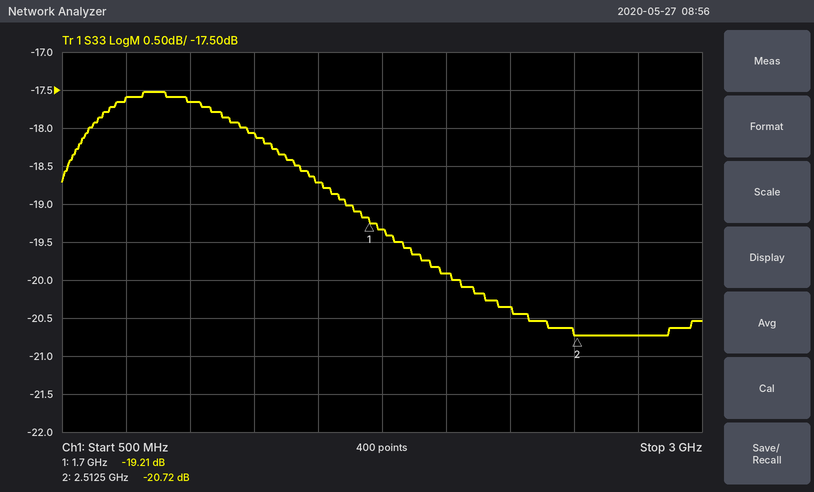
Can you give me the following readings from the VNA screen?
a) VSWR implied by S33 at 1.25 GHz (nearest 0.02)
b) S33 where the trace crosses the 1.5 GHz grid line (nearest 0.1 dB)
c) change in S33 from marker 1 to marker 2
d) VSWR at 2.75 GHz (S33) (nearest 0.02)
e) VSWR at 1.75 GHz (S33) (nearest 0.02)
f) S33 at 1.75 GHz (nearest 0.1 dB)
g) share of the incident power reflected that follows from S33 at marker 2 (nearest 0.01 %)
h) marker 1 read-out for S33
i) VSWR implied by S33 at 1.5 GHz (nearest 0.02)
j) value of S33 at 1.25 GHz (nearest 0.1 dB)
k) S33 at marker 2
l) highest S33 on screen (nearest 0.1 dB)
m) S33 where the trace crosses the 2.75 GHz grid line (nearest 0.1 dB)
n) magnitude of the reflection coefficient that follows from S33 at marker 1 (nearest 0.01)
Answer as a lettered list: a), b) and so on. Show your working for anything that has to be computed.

a) |Γ| = 10^(-18.1/20) = 0.1245; VSWR = (1 + 0.1245)/(1 − 0.1245) ≈ 1.28
b) -18.7 dB
c) -20.72 − (-19.21) = -1.51 dB
d) |Γ| = 10^(-20.7/20) = 0.0923; VSWR = (1 + 0.0923)/(1 − 0.0923) ≈ 1.20
e) |Γ| = 10^(-19.3/20) = 0.1084; VSWR = (1 + 0.1084)/(1 − 0.1084) ≈ 1.24
f) -19.3 dB
g) 10^(-20.72/10) ≈ 0.85 %
h) -19.21 dB
i) |Γ| = 10^(-18.7/20) = 0.1161; VSWR = (1 + 0.1161)/(1 − 0.1161) ≈ 1.26
j) -18.1 dB
k) -20.72 dB
l) -17.5 dB
m) -20.7 dB
n) 10^(-19.21/20) ≈ 0.11
